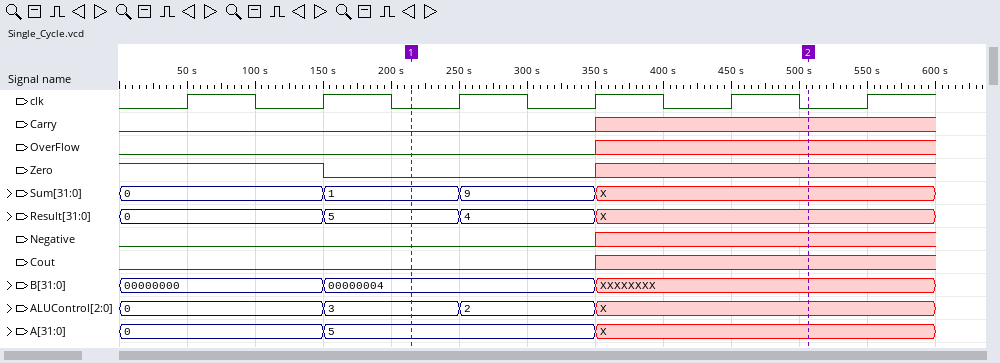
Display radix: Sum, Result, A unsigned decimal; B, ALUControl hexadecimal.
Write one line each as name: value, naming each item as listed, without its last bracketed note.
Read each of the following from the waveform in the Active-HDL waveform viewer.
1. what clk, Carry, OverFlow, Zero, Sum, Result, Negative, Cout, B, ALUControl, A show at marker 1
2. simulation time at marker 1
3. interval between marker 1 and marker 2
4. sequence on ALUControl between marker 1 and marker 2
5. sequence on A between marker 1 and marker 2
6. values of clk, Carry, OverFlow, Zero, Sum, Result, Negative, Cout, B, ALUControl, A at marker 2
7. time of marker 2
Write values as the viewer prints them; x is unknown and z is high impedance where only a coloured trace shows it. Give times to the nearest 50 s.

what clk, Carry, OverFlow, Zero, Sum, Result, Negative, Cout, B, ALUControl, A show at marker 1: clk=0, Carry=0, OverFlow=0, Zero=0, Sum=1, Result=5, Negative=0, Cout=0, B=00000004, ALUControl=3, A=5
simulation time at marker 1: 200 s
interval between marker 1 and marker 2: 300 s
sequence on ALUControl between marker 1 and marker 2: 3, 2, X
sequence on A between marker 1 and marker 2: 5, X
values of clk, Carry, OverFlow, Zero, Sum, Result, Negative, Cout, B, ALUControl, A at marker 2: clk=0, Carry=x, OverFlow=x, Zero=x, Sum=X, Result=X, Negative=x, Cout=x, B=XXXXXXXX, ALUControl=X, A=X
time of marker 2: 500 s
